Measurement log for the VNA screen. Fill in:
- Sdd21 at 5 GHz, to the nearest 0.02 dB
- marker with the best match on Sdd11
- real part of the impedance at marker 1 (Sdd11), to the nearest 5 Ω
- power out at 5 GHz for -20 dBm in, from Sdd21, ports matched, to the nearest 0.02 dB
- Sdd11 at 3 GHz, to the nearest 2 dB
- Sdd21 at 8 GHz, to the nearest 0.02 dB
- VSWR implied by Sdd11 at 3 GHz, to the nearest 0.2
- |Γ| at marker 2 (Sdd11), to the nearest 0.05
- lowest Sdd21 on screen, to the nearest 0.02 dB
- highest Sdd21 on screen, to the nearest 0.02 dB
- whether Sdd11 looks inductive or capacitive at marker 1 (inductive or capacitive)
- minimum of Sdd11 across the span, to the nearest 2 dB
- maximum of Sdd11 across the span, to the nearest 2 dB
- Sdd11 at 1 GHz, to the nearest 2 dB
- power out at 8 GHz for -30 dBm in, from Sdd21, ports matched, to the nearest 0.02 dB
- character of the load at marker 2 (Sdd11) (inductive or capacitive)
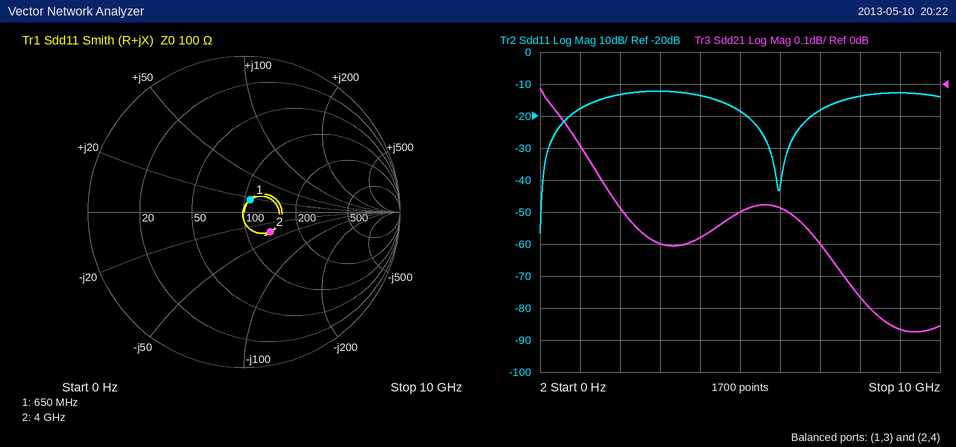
-0.40 dB
marker 1
105 Ω
-20.40 dBm
-12 dB
-0.66 dB
1.6
0.20
-0.78 dB
-0.02 dB
inductive
-56 dB
-12 dB
-18 dB
-30.66 dBm
capacitive
